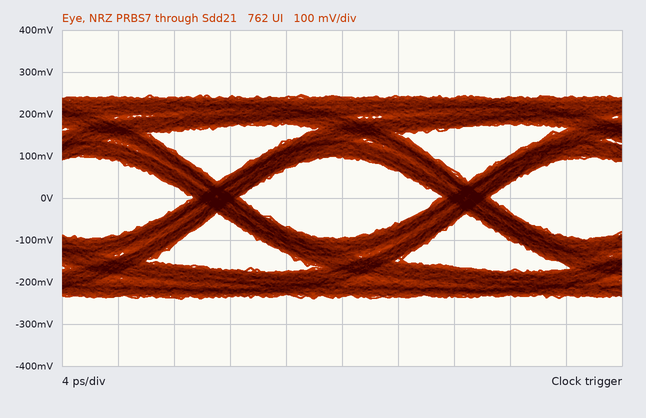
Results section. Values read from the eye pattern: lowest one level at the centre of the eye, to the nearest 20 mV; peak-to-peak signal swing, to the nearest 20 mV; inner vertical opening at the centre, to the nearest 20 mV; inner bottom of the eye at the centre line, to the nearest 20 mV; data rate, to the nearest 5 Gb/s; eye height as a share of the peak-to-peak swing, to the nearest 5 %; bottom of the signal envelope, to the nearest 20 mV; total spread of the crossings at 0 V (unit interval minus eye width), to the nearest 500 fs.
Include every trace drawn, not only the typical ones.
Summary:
100 mV
480 mV
200 mV
-100 mV
55 Gb/s
40 %
-240 mV
3.5 ps
